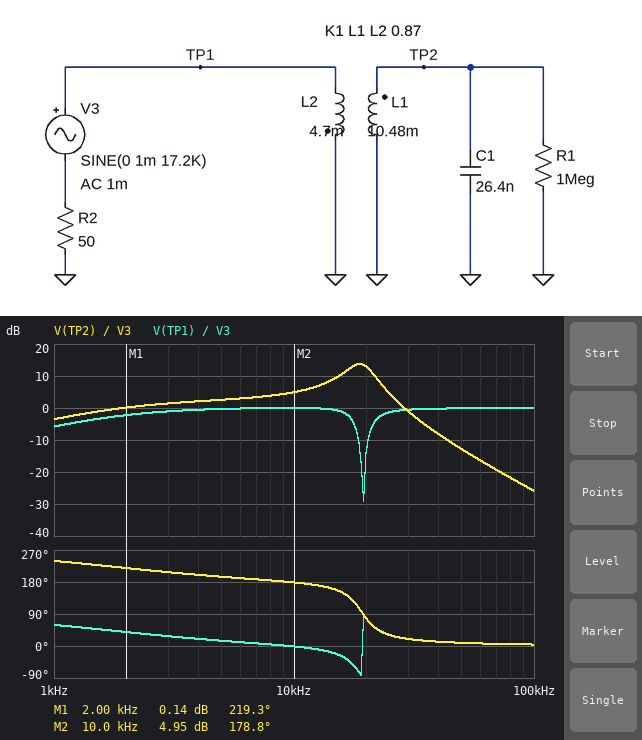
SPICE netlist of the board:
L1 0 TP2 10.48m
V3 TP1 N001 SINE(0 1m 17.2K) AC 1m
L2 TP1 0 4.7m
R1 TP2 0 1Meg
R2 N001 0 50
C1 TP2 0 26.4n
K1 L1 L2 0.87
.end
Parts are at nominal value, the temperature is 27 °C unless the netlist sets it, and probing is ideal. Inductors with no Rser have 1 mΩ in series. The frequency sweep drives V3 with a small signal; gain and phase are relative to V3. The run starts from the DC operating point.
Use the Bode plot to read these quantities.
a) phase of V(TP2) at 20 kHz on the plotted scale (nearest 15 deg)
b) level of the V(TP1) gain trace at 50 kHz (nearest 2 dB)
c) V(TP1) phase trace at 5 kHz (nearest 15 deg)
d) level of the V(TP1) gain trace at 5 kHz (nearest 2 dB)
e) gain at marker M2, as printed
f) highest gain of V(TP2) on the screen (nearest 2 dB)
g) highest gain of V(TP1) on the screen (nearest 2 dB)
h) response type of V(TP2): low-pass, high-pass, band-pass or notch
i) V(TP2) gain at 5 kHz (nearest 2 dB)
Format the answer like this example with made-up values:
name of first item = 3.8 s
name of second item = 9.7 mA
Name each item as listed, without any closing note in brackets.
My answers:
phase of V(TP2) at 20 kHz on the plotted scale = 75 deg
level of the V(TP1) gain trace at 50 kHz = 0 dB
V(TP1) phase trace at 5 kHz = 15 deg
level of the V(TP1) gain trace at 5 kHz = 0 dB
gain at marker M2, as printed = 4.95 dB
highest gain of V(TP2) on the screen = 14 dB
highest gain of V(TP1) on the screen = 0 dB
response type of V(TP2): low-pass, high-pass, band-pass or notch = band-pass
V(TP2) gain at 5 kHz = 2 dB
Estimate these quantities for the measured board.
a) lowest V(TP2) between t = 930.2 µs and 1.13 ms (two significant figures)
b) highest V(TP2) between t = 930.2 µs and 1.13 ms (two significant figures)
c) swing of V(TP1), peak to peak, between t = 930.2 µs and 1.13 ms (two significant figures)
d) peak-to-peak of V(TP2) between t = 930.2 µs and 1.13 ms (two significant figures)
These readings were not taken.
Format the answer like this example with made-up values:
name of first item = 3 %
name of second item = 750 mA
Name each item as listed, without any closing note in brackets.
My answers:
lowest V(TP2) between t = 930.2 µs and 1.13 ms = -4.2 mV
highest V(TP2) between t = 930.2 µs and 1.13 ms = 4.2 mV
swing of V(TP1), peak to peak, between t = 930.2 µs and 1.13 ms = 1.4 mV
peak-to-peak of V(TP2) between t = 930.2 µs and 1.13 ms = 8.5 mV
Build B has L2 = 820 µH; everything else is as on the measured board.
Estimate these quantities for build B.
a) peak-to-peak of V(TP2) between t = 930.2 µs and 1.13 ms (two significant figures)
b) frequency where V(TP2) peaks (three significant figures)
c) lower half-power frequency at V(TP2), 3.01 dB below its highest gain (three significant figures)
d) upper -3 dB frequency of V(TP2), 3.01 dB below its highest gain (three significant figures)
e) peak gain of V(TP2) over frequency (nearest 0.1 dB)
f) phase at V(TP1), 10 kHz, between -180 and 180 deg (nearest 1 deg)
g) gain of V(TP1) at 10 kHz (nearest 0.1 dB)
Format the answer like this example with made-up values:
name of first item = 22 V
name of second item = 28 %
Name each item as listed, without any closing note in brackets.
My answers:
peak-to-peak of V(TP2) between t = 930.2 µs and 1.13 ms = 4.9 mV
frequency where V(TP2) peaks = 10.6 kHz
lower half-power frequency at V(TP2), 3.01 dB below its highest gain = 7.23 kHz
upper -3 dB frequency of V(TP2), 3.01 dB below its highest gain = 15.1 kHz
peak gain of V(TP2) over frequency = 12.6 dB
phase at V(TP1), 10 kHz, between -180 and 180 deg = -7 deg
gain of V(TP1) at 10 kHz = -0.1 dB
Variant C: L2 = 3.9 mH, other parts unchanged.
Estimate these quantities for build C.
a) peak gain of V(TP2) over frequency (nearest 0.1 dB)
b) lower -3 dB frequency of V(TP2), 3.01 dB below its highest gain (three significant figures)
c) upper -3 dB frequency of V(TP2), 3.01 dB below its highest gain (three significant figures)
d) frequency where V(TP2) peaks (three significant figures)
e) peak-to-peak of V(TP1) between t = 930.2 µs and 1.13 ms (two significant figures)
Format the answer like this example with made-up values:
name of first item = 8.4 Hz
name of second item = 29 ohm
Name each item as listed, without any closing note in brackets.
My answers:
peak gain of V(TP2) over frequency = 13.1 dB
lower -3 dB frequency of V(TP2), 3.01 dB below its highest gain = 15.0 kHz
upper -3 dB frequency of V(TP2), 3.01 dB below its highest gain = 21.5 kHz
frequency where V(TP2) peaks = 18.5 kHz
peak-to-peak of V(TP1) between t = 930.2 µs and 1.13 ms = 1.3 mV
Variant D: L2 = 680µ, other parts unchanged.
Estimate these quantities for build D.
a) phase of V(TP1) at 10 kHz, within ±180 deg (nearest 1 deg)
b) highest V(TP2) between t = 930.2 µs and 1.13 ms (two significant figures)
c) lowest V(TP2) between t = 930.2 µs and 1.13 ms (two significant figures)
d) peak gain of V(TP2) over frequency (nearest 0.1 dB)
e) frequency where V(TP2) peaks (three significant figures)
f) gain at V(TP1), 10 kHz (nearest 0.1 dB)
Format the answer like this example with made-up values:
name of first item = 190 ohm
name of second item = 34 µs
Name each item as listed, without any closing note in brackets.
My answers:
phase of V(TP1) at 10 kHz, within ±180 deg = -8 deg
highest V(TP2) between t = 930.2 µs and 1.13 ms = 2.2 mV
lowest V(TP2) between t = 930.2 µs and 1.13 ms = -2.2 mV
peak gain of V(TP2) over frequency = 13.3 dB
frequency where V(TP2) peaks = 10.2 kHz
gain at V(TP1), 10 kHz = -0.1 dB
